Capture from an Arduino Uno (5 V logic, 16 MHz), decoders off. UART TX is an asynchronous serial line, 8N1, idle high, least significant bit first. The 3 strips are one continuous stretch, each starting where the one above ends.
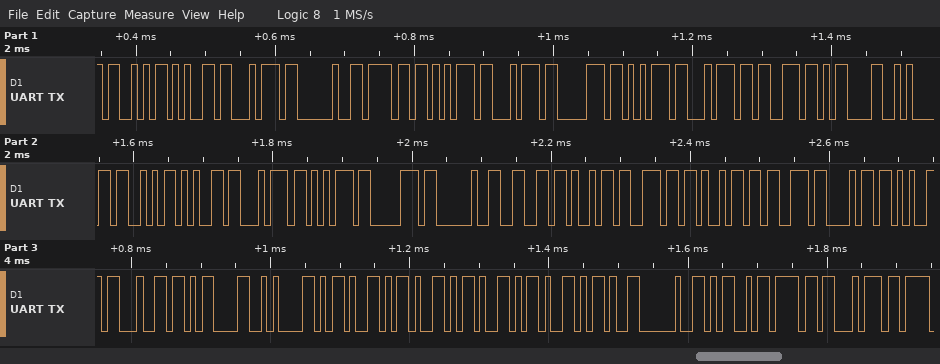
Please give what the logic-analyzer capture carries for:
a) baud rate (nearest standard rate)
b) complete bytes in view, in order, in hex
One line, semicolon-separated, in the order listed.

115200 baud; 53 65 74 20 6F 75 74 70 75 74 73 0D 0A 53 65 74 75 70 20 66 69 6E 69 73 68 65 64 0D 0A 2D 2D 2D 2D 2D 20 4D 6F 74
